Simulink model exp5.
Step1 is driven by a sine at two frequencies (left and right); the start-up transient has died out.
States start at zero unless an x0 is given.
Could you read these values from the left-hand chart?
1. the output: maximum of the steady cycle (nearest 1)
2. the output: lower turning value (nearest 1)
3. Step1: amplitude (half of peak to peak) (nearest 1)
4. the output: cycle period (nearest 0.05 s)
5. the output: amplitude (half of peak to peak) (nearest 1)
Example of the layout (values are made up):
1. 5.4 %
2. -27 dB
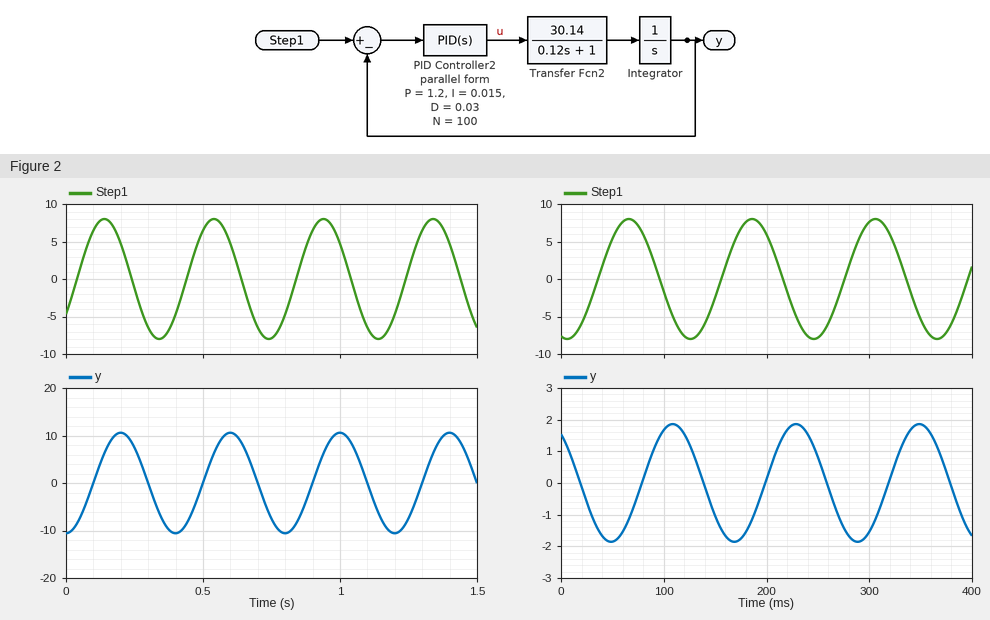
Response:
1. 11
2. -11
3. 8
4. 0.40 s
5. 11
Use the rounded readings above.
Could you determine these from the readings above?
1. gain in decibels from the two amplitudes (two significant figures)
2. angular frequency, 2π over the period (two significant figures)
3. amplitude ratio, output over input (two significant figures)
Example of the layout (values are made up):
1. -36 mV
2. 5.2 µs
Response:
1. 2.8 dB
2. 16 rad/s
3. 1.4
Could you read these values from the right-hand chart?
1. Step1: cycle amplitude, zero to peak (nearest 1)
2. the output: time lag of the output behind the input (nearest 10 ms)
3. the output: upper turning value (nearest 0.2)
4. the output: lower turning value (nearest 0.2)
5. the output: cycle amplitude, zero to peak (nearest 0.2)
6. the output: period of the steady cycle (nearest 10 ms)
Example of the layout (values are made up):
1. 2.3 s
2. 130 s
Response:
1. 8
2. 40 ms
3. 1.8
4. -1.8
5. 1.8
6. 120 ms
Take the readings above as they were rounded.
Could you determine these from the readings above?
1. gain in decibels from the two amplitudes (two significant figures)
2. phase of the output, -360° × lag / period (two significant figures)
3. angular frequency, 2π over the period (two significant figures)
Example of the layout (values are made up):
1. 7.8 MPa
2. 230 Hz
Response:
1. -13 dB
2. -120°
3. 0.052 rad/ms
